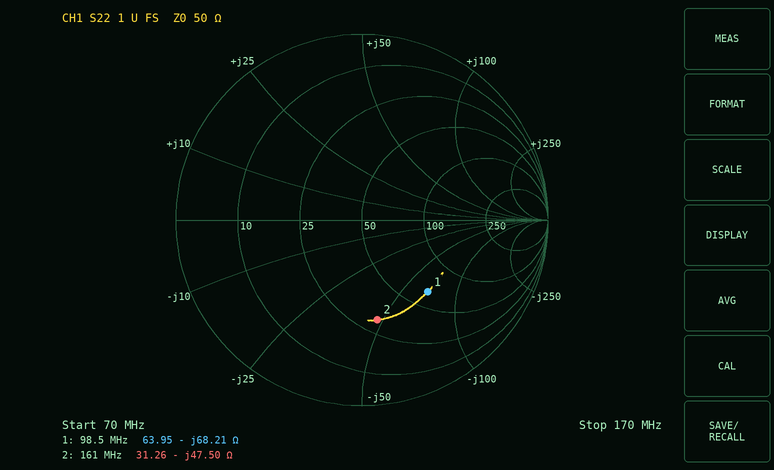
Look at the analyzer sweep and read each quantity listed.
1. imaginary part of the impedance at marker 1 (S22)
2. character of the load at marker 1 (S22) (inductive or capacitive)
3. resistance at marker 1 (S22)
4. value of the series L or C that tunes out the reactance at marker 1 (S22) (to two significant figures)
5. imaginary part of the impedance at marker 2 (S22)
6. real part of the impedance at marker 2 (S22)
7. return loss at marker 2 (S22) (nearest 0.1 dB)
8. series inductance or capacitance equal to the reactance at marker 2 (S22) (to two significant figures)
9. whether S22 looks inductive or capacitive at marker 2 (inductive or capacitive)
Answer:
-68.21 Ω
capacitive
63.95 Ω
110 nH
-47.50 Ω
31.26 Ω
5.3 dB
21 pF
capacitive
